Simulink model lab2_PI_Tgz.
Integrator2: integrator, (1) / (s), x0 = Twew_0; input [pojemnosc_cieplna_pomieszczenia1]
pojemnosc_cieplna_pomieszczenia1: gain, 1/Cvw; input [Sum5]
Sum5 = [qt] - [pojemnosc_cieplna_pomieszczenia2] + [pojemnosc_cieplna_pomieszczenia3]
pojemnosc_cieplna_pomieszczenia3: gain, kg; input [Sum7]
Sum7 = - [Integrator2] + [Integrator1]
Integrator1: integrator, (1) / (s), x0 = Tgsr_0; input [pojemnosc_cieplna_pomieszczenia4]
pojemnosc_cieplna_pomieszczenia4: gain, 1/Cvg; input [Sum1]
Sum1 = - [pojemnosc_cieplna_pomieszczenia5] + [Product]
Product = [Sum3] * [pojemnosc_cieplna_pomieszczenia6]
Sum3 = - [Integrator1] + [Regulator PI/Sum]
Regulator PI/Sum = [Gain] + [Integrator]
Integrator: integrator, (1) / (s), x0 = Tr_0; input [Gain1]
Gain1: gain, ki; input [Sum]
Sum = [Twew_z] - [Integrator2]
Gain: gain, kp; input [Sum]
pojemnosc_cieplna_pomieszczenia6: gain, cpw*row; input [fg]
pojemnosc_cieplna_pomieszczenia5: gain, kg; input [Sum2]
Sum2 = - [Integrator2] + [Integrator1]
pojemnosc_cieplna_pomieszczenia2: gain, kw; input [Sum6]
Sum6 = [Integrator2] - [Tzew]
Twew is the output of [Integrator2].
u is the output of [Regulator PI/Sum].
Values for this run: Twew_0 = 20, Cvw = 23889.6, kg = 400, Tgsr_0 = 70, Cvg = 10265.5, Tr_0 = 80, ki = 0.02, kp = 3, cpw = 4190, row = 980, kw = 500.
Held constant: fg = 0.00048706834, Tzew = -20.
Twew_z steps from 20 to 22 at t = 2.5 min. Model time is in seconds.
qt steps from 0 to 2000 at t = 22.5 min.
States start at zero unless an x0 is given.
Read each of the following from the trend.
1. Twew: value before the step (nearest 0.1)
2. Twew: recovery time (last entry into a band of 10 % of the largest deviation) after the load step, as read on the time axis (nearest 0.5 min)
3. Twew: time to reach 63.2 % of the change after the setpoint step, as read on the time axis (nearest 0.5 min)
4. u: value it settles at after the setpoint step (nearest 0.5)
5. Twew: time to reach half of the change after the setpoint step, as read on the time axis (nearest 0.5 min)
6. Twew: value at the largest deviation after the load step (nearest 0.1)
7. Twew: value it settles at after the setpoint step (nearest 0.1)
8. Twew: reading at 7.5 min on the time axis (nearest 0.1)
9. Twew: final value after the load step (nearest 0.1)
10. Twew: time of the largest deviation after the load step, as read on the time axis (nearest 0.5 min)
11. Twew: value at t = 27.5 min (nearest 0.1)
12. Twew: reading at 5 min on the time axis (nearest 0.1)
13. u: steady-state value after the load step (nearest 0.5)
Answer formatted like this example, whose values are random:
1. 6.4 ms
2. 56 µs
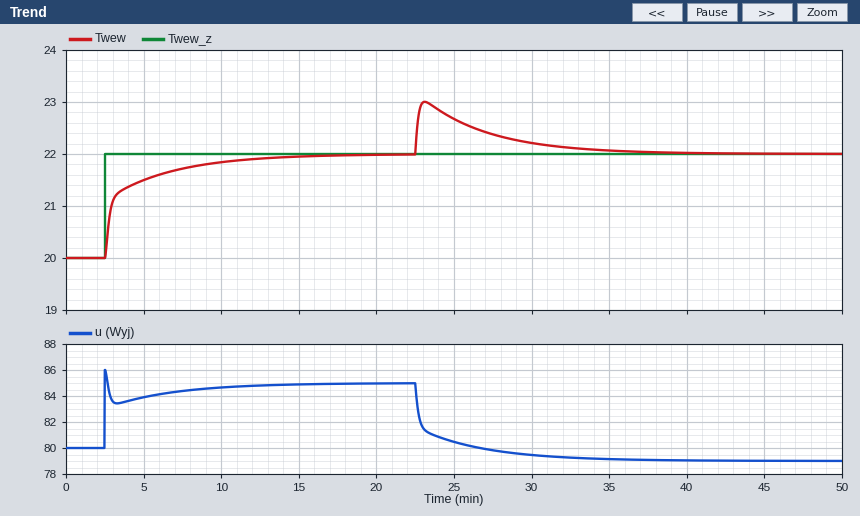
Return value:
1. 20.0
2. 33.0 min
3. 3.5 min
4. 85.0
5. 3.0 min
6. 23.0
7. 22.0
8. 21.7
9. 22.0
10. 23.0 min
11. 22.4
12. 21.5
13. 79.0
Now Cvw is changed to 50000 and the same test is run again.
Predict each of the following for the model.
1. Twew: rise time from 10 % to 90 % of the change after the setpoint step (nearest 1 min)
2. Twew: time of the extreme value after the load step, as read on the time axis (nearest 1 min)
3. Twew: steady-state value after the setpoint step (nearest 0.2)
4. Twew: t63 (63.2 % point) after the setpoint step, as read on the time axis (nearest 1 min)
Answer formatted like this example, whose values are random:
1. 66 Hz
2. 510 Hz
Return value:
1. 6 min
2. 24 min
3. 22.0
4. 4 min
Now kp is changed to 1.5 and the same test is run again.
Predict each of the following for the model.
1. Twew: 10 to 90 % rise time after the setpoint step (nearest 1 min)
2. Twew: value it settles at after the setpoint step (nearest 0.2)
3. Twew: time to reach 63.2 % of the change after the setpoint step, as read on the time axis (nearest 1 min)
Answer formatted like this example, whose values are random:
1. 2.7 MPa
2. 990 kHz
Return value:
1. 5 min
2. 22.0
3. 4 min
